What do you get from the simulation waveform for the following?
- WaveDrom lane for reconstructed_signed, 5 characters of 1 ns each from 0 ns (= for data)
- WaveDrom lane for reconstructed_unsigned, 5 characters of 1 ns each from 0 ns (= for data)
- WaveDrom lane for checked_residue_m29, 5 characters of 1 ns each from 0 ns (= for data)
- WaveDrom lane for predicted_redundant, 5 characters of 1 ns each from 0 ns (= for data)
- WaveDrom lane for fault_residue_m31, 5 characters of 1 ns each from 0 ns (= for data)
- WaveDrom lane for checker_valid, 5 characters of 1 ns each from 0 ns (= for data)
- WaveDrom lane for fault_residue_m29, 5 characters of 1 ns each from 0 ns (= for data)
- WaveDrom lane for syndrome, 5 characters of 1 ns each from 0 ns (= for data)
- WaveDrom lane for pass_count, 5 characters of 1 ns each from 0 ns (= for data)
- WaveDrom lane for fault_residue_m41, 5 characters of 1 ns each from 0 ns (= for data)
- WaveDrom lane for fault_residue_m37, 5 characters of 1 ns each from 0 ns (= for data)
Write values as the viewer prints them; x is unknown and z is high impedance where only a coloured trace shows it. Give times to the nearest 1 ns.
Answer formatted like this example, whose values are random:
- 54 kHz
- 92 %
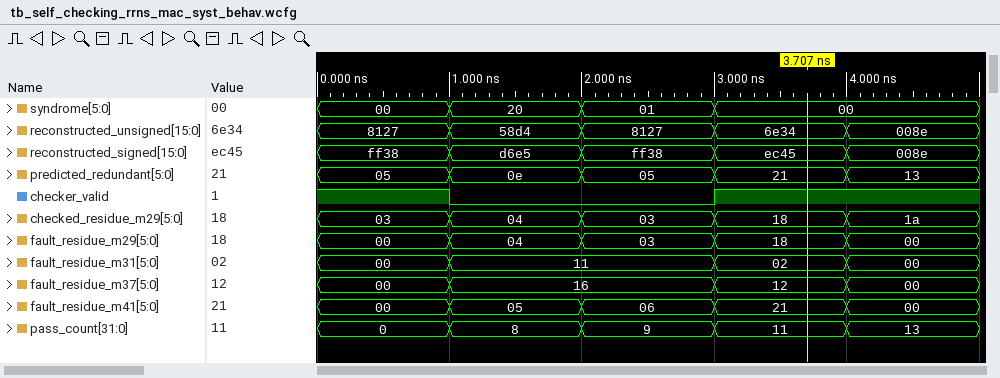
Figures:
- {name: 'reconstructed_signed', wave: '=====', data: 'ff38 d6e5 ff38 ec45 008e'}
- {name: 'reconstructed_unsigned', wave: '=====', data: '8127 58d4 8127 6e34 008e'}
- {name: 'checked_residue_m29', wave: '=====', data: '03 04 03 18 1a'}
- {name: 'predicted_redundant', wave: '=====', data: '05 0e 05 21 13'}
- {name: 'fault_residue_m31', wave: '==.==', data: '00 11 02 00'}
- {name: 'checker_valid', wave: '10.1.'}
- {name: 'fault_residue_m29', wave: '=====', data: '00 04 03 18 00'}
- {name: 'syndrome', wave: '====.', data: '00 20 01 00'}
- {name: 'pass_count', wave: '=====', data: '0 8 9 11 13'}
- {name: 'fault_residue_m41', wave: '=====', data: '00 05 06 21 00'}
- {name: 'fault_residue_m37', wave: '==.==', data: '00 16 12 00'}
